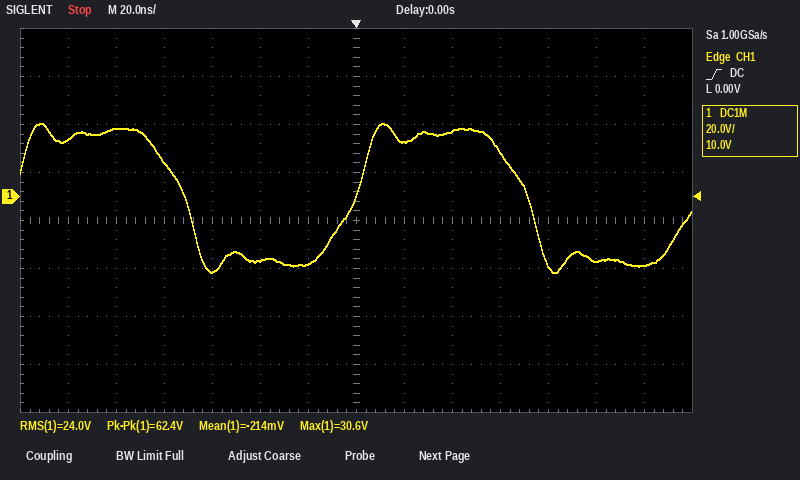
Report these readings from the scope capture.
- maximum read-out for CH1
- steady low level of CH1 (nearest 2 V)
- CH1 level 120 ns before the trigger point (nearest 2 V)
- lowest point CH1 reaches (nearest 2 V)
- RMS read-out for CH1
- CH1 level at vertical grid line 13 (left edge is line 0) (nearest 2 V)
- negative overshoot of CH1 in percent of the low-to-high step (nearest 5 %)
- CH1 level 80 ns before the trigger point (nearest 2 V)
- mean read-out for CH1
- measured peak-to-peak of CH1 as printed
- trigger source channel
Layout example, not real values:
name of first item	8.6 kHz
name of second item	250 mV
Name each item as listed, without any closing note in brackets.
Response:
maximum read-out for CH1	30.6 V
steady low level of CH1	-28 V
CH1 level 120 ns before the trigger point	24 V
lowest point CH1 reaches	-32 V
RMS read-out for CH1	24.0 V
CH1 level at vertical grid line 13 (left edge is line 0)	-28 V
negative overshoot of CH1 in percent of the low-to-high step	10 %
CH1 level 80 ns before the trigger point	14 V
mean read-out for CH1	-214 mV
measured peak-to-peak of CH1 as printed	62.4 V
trigger source channel	CH1
